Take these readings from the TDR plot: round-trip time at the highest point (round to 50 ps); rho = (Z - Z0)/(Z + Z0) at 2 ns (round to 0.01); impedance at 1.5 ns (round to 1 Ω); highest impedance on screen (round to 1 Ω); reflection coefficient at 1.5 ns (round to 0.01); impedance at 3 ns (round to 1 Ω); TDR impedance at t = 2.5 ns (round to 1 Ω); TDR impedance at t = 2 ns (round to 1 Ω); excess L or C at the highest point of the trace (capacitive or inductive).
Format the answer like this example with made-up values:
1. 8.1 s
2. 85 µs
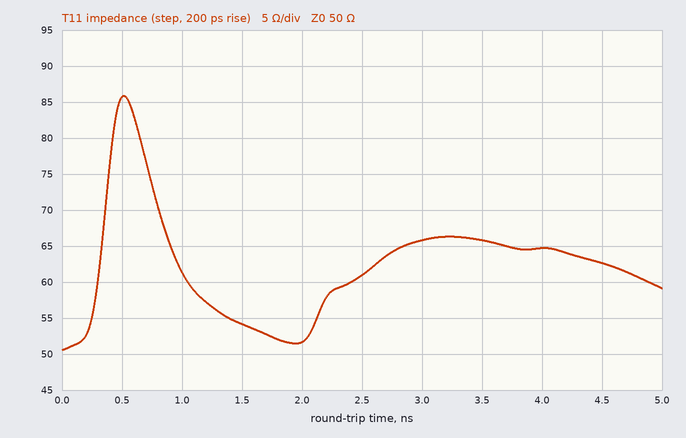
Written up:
1. 500 ps
2. +0.02
3. 54 Ω
4. 86 Ω
5. +0.04
6. 66 Ω
7. 61 Ω
8. 52 Ω
9. inductive
